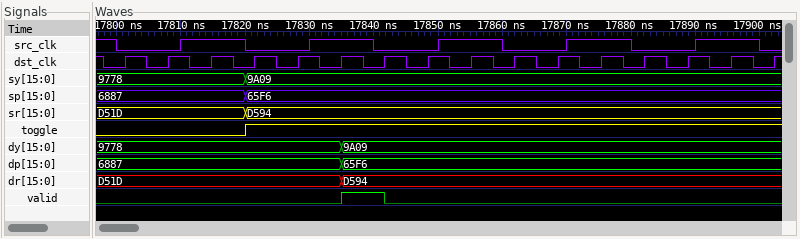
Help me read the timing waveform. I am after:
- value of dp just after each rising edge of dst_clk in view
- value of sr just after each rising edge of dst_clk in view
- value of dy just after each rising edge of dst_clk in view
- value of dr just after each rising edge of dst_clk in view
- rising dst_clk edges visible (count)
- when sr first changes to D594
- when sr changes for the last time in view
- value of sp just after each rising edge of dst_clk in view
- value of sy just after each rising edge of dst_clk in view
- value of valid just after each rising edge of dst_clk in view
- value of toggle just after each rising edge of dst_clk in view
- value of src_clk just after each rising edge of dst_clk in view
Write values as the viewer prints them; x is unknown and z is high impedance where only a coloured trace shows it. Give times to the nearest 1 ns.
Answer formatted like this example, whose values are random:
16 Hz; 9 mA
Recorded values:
6887, 6887, 6887, 6887, 6887, 65F6, 65F6, 65F6, 65F6, 65F6, 65F6, 65F6, 65F6, 65F6, 65F6, 65F6; D51D, D51D, D51D, D594, D594, D594, D594, D594, D594, D594, D594, D594, D594, D594, D594, D594; 9778, 9778, 9778, 9778, 9778, 9A09, 9A09, 9A09, 9A09, 9A09, 9A09, 9A09, 9A09, 9A09, 9A09, 9A09; D51D, D51D, D51D, D51D, D51D, D594, D594, D594, D594, D594, D594, D594, D594, D594, D594, D594; 16; 17820 ns; 17820 ns; 6887, 6887, 6887, 65F6, 65F6, 65F6, 65F6, 65F6, 65F6, 65F6, 65F6, 65F6, 65F6, 65F6, 65F6, 65F6; 9778, 9778, 9778, 9A09, 9A09, 9A09, 9A09, 9A09, 9A09, 9A09, 9A09, 9A09, 9A09, 9A09, 9A09, 9A09; 0 0 0 0 0 1 0 0 0 0 0 0 0 0 0 0; 0 0 0 1 1 1 1 1 1 1 1 1 1 1 1 1; 0 0 1 0 0 1 0 0 1 0 0 1 0 0 1 0
